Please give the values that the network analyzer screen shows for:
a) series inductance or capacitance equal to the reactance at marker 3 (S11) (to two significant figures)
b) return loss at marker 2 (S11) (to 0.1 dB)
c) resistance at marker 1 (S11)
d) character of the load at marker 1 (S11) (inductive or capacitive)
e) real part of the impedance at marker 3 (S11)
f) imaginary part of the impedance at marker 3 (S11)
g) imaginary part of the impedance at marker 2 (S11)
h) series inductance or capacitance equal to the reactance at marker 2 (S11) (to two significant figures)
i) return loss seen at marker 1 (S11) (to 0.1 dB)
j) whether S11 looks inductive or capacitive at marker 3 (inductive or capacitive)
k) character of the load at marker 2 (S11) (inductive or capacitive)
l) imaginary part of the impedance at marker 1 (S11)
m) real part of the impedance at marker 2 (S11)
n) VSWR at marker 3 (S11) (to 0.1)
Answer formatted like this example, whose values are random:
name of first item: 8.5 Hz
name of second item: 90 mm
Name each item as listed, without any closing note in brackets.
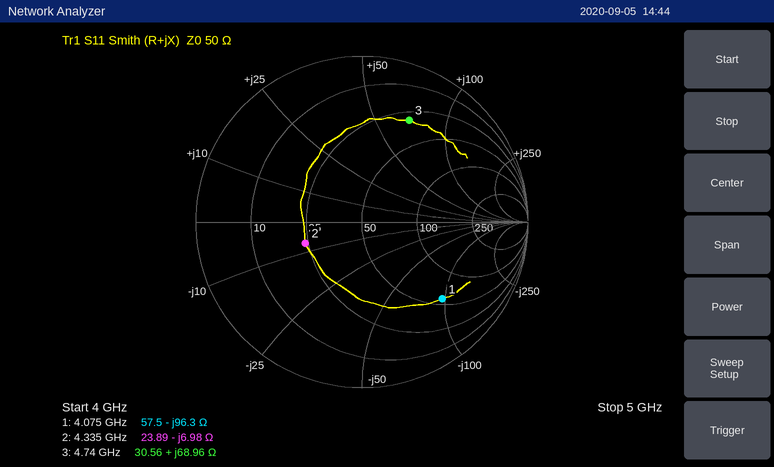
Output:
series inductance or capacitance equal to the reactance at marker 3 (S11): 2.3 nH
return loss at marker 2 (S11): 8.8 dB
resistance at marker 1: 57.5 Ω
character of the load at marker 1 (S11): capacitive
real part of the impedance at marker 3: 30.56 Ω
imaginary part of the impedance at marker 3: +68.96 Ω
imaginary part of the impedance at marker 2: -6.98 Ω
series inductance or capacitance equal to the reactance at marker 2 (S11): 5.3 pF
return loss seen at marker 1 (S11): 3.5 dB
whether S11 looks inductive or capacitive at marker 3: inductive
character of the load at marker 2 (S11): capacitive
imaginary part of the impedance at marker 1: -96.3 Ω
real part of the impedance at marker 2: 23.89 Ω
VSWR at marker 3 (S11): 5.2
